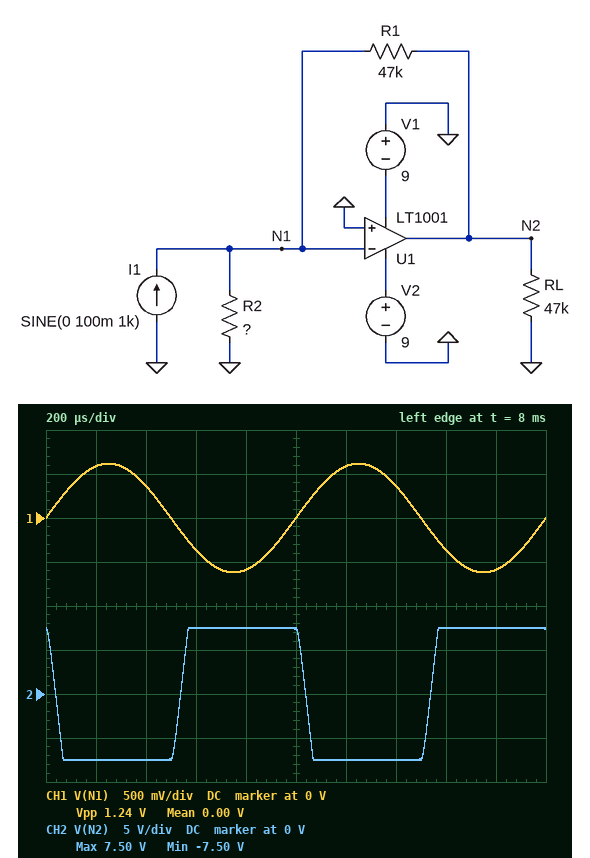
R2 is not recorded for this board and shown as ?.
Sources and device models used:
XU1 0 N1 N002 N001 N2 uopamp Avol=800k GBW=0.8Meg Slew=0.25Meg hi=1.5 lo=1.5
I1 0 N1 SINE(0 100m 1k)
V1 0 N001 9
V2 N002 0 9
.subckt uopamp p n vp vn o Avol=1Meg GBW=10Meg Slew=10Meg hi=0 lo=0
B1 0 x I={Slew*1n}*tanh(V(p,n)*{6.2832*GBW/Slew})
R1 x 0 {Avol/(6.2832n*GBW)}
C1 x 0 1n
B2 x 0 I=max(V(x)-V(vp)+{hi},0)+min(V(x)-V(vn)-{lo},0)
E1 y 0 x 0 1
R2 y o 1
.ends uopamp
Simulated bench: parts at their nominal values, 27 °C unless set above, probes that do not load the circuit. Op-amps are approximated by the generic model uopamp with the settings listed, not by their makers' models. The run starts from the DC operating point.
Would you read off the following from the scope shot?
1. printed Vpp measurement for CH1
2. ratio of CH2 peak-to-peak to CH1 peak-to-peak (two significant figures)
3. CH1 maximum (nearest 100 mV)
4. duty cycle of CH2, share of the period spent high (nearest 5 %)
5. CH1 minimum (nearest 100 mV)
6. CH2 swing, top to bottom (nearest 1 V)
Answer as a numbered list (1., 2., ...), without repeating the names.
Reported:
1. 1.24 V
2. 12
3. 600 mV
4. 50 %
5. -600 mV
6. 15 V
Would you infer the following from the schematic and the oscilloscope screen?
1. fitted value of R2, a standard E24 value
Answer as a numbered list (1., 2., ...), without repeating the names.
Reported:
1. 6.2 Ω
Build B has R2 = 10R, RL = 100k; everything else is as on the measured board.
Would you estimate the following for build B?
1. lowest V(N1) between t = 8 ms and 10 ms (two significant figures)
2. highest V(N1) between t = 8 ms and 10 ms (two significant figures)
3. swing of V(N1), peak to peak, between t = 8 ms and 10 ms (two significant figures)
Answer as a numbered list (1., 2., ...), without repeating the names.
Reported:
1. -1.0 V
2. 1.0 V
3. 2.0 V
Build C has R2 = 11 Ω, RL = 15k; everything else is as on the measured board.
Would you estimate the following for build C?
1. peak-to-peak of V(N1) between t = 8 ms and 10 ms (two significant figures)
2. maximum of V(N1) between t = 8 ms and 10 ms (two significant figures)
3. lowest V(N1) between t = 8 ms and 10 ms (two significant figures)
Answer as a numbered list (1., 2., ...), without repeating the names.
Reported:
1. 2.2 V
2. 1.1 V
3. -1.1 V
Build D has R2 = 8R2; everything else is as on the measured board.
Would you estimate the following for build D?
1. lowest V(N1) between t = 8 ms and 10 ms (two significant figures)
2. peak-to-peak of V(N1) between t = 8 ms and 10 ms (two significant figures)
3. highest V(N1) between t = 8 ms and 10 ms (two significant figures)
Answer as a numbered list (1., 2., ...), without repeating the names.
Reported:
1. -820 mV
2. 1.6 V
3. 820 mV
